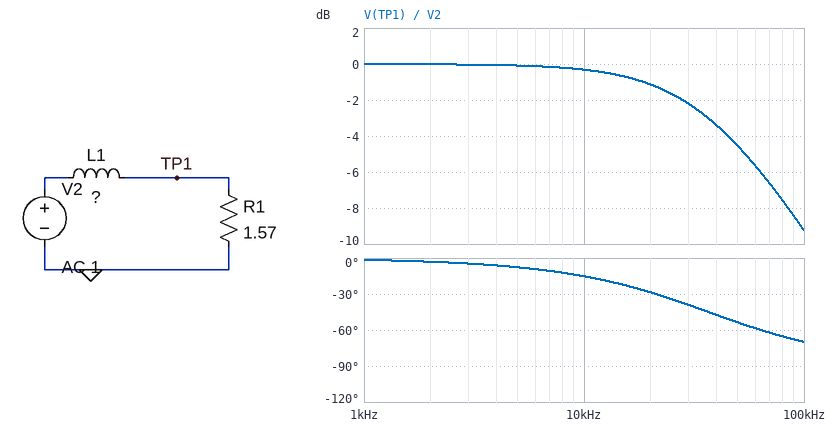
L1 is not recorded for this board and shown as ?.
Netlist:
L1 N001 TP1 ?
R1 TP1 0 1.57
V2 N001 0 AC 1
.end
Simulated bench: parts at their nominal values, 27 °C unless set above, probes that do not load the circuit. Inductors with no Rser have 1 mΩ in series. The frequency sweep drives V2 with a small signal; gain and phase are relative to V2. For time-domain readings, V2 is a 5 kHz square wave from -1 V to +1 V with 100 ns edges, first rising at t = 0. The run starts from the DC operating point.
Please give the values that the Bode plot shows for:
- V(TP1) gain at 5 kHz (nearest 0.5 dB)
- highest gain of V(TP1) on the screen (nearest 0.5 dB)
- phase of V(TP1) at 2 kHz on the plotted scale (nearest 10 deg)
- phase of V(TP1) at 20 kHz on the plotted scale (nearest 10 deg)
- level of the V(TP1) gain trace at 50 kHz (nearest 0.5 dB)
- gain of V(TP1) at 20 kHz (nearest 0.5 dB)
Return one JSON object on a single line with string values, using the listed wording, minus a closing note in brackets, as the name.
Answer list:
{"V(TP1) gain at 5 kHz": "0 dB", "highest gain of V(TP1) on the screen": "0 dB", "phase of V(TP1) at 2 kHz on the plotted scale": "0 deg", "phase of V(TP1) at 20 kHz on the plotted scale": "-30 deg", "level of the V(TP1) gain trace at 50 kHz": "-4.5 dB", "gain of V(TP1) at 20 kHz": "-1.0 dB"}
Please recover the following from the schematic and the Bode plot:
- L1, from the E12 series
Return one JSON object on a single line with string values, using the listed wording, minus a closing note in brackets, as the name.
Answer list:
{"L1, from the E12 series": "6.8 µH"}
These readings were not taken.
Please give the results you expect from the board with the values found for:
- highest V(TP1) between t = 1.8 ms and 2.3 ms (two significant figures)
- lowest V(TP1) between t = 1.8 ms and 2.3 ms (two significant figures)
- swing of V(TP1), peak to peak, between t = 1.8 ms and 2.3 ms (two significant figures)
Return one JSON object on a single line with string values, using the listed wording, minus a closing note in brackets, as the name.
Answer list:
{"highest V(TP1) between t = 1.8 ms and 2.3 ms": "1.0 V", "lowest V(TP1) between t = 1.8 ms and 2.3 ms": "-1.0 V", "swing of V(TP1), peak to peak, between t = 1.8 ms and 2.3 ms": "2.0 V"}
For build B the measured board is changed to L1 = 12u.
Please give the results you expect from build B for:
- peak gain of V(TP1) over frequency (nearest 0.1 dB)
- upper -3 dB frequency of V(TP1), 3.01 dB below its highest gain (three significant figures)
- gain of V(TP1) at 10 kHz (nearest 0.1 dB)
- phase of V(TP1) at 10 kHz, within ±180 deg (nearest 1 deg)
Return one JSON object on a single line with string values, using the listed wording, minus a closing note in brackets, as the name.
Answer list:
{"peak gain of V(TP1) over frequency": "0 dB", "upper -3 dB frequency of V(TP1), 3.01 dB below its highest gain": "20.8 kHz", "gain of V(TP1) at 10 kHz": "-0.9 dB", "phase of V(TP1) at 10 kHz, within ±180 deg": "-26 deg"}
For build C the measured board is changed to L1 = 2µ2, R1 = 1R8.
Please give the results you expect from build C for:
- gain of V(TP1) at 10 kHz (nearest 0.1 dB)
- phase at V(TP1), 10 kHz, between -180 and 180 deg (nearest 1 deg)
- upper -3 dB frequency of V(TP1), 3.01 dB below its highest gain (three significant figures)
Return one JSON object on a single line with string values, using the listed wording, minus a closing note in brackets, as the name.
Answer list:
{"gain of V(TP1) at 10 kHz": "0 dB", "phase at V(TP1), 10 kHz, between -180 and 180 deg": "-4 deg", "upper -3 dB frequency of V(TP1), 3.01 dB below its highest gain": "130 kHz"}
